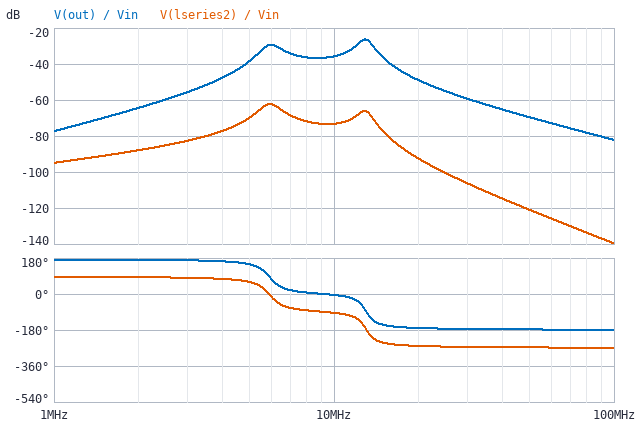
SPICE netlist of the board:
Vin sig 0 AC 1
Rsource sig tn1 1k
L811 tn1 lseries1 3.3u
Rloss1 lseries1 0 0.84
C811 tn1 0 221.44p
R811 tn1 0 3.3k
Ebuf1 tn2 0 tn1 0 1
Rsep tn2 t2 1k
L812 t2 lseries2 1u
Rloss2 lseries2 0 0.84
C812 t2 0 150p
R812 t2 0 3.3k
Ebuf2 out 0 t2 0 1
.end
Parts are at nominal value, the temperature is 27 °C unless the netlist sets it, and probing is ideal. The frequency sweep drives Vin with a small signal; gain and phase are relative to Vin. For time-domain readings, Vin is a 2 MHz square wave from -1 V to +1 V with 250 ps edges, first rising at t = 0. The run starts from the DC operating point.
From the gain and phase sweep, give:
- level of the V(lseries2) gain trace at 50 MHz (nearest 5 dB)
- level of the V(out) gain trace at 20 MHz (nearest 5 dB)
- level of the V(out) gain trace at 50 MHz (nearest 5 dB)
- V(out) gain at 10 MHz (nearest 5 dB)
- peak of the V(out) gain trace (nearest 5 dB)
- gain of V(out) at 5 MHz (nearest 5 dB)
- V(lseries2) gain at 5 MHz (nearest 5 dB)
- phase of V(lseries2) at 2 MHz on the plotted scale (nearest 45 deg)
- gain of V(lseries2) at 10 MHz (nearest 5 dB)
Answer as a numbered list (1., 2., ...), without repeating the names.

1. -120 dB
2. -50 dB
3. -70 dB
4. -35 dB
5. -25 dB
6. -40 dB
7. -70 dB
8. 90 deg
9. -75 dB
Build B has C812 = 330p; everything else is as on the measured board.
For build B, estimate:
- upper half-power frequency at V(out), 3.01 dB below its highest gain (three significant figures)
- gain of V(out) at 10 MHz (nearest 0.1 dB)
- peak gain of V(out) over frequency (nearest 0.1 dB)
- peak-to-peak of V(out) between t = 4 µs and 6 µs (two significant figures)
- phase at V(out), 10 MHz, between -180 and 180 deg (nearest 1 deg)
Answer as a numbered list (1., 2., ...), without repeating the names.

1. 9.08 MHz
2. -33.3 dB
3. -20.6 dB
4. 51 mV
5. -154 deg
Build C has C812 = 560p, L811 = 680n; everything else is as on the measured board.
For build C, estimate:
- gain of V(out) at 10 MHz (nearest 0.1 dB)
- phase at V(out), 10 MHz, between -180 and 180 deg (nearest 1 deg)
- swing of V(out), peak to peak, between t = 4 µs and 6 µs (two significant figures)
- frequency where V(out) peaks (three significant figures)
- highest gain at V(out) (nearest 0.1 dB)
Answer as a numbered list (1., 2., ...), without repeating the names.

1. -45.4 dB
2. -6 deg
3. 9.1 mV
4. 6.75 MHz
5. -33.1 dB
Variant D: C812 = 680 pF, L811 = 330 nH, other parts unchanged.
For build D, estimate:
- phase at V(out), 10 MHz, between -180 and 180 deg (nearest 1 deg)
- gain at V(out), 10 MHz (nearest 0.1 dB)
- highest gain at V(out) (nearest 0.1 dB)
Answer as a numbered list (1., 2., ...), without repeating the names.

1. -2 deg
2. -59.3 dB
3. -42.4 dB
